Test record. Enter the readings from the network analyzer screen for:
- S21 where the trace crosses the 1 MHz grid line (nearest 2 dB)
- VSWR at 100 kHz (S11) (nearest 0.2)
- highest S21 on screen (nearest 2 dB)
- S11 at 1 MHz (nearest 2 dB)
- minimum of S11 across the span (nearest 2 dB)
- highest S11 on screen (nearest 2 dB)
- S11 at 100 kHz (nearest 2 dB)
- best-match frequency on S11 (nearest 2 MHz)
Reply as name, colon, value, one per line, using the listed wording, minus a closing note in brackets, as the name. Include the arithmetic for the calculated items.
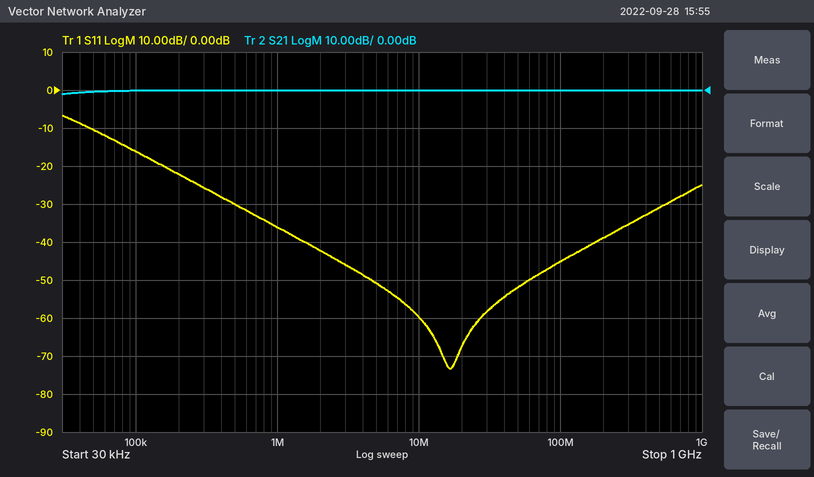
S21 where the trace crosses the 1 MHz grid line: 0 dB
VSWR at 100 kHz (S11): |Γ| = 10^(-16/20) = 0.1585; VSWR = (1 + 0.1585)/(1 − 0.1585) ≈ 1.4
highest S21 on screen: 0 dB
S11 at 1 MHz: -36 dB
minimum of S11 across the span: -74 dB
highest S11 on screen: -6 dB
S11 at 100 kHz: -16 dB
best-match frequency on S11: 16 MHz
